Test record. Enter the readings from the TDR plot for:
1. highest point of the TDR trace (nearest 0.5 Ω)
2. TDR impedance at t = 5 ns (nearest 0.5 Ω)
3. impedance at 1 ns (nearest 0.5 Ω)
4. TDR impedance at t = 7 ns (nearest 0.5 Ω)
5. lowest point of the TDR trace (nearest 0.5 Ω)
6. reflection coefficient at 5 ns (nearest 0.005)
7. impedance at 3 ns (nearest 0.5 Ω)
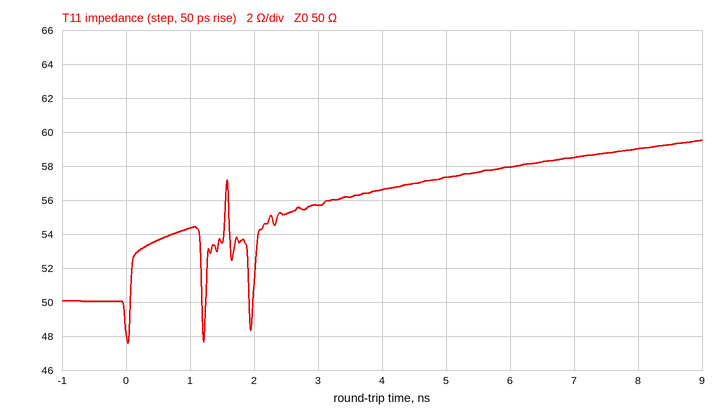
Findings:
59.5 Ω
57.5 Ω
54.5 Ω
58.5 Ω
47.5 Ω
+0.070
55.5 Ω
